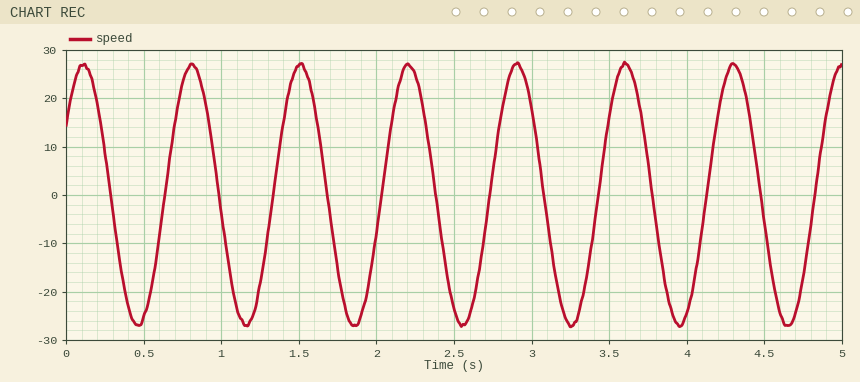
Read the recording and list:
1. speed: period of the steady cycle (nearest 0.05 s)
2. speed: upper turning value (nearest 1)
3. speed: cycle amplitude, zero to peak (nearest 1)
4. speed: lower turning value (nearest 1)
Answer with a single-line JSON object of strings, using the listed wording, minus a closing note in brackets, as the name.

{"speed: period of the steady cycle": "0.70 s", "speed: upper turning value": "27", "speed: cycle amplitude, zero to peak": "27", "speed: lower turning value": "-27"}
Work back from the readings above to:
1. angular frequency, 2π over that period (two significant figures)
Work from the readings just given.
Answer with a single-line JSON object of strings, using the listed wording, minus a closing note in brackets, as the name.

{"angular frequency, 2π over that period": "9.0 rad/s"}
